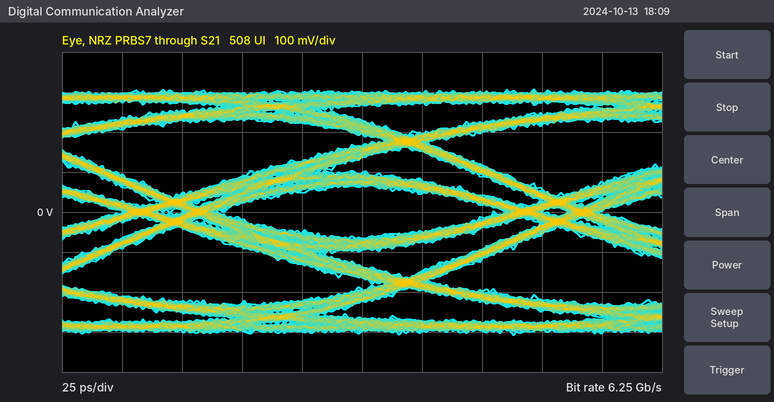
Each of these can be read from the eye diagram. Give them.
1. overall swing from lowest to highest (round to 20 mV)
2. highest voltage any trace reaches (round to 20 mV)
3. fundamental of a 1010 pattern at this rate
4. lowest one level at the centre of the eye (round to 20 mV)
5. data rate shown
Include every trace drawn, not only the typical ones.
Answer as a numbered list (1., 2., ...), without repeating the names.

1. 620 mV
2. 300 mV
3. 3.125 GHz
4. 60 mV
5. 6.25 Gb/s
